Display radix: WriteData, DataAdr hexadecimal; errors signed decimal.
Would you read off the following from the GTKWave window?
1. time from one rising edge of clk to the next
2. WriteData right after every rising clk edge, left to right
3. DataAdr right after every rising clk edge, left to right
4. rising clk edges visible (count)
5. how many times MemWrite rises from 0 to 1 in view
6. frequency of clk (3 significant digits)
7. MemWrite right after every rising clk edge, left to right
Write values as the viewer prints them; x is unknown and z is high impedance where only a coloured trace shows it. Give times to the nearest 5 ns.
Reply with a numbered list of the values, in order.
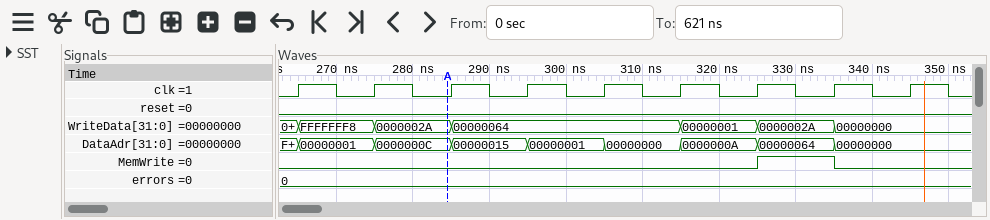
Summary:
1. 10 ns
2. FFFFFFF8, 0000002A, 00000064, 00000064, 00000064, 00000001, 0000002A, 00000000, 00000000
3. 00000001, 0000000C, 00000015, 00000001, 00000000, 0000000A, 00000064, 00000000, 00000000
4. 9
5. 1
6. 100 MHz
7. 0 0 0 0 0 0 1 0 0
